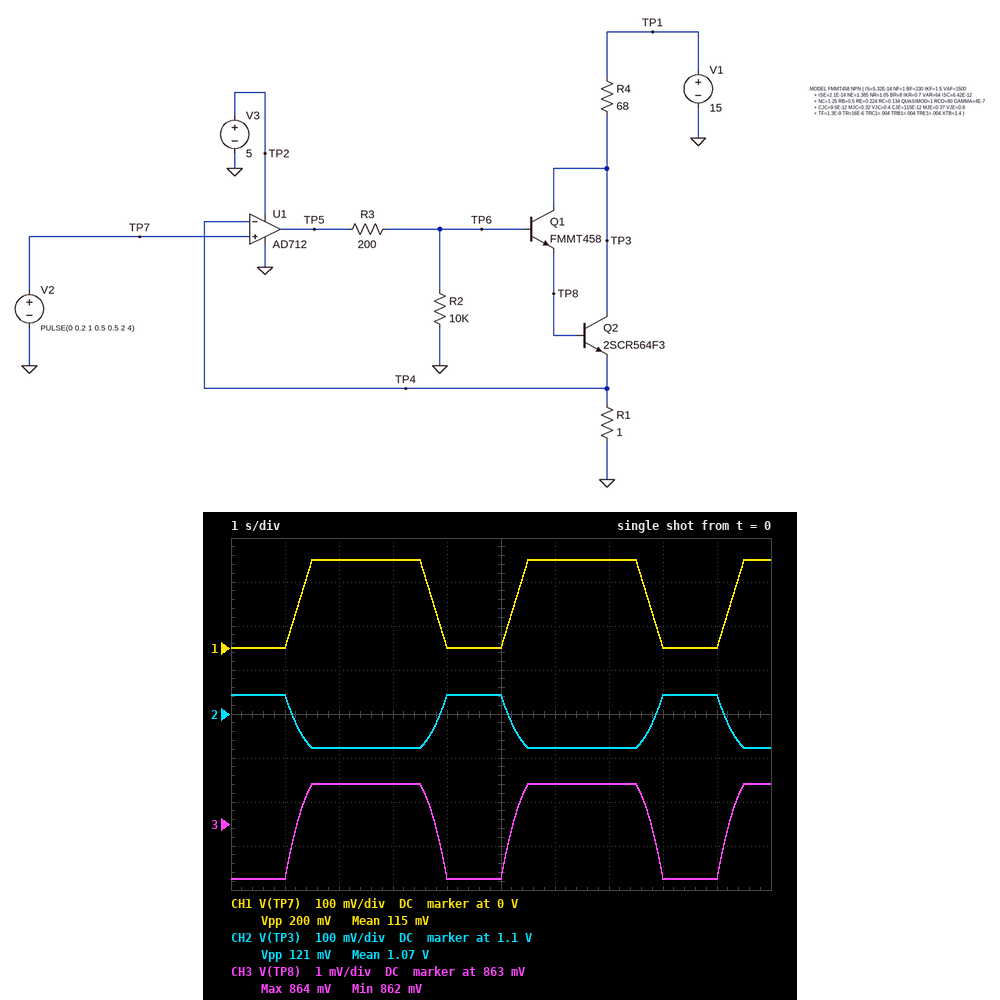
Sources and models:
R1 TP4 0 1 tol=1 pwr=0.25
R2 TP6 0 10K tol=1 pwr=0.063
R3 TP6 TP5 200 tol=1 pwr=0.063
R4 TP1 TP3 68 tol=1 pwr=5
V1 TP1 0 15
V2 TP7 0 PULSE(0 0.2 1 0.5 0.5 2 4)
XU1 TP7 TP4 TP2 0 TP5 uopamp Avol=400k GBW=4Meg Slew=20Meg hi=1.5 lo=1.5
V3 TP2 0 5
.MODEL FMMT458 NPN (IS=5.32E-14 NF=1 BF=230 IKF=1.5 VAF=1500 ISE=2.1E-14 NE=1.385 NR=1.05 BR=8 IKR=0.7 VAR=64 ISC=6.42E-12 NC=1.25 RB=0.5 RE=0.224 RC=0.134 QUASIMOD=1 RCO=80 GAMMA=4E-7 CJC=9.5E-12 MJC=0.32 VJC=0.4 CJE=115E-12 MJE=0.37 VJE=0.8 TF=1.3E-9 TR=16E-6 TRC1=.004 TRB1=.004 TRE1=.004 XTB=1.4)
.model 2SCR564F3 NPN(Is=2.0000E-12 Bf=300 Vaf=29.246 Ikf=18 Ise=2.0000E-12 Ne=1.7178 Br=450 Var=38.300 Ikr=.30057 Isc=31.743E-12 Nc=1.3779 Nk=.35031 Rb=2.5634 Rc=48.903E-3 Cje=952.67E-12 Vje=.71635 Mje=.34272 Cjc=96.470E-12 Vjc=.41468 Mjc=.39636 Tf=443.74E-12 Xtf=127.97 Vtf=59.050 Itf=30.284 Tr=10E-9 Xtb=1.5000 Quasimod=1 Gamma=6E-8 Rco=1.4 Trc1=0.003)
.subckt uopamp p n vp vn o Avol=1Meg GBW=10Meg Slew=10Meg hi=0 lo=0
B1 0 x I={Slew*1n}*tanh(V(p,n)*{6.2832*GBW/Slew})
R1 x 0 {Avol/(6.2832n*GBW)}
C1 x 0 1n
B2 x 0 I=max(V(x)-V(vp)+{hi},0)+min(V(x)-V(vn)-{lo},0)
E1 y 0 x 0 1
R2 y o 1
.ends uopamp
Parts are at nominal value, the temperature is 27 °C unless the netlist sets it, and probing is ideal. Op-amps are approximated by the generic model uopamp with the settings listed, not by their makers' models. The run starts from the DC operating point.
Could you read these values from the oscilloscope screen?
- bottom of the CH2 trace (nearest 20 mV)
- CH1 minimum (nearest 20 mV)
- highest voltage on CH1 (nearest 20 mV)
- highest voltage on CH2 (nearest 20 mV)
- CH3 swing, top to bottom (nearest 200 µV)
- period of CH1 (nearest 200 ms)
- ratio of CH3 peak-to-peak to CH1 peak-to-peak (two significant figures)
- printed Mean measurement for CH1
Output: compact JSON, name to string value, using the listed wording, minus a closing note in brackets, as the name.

{"bottom of the CH2 trace": "1.02 V", "CH1 minimum": "0 V", "highest voltage on CH1": "200 mV", "highest voltage on CH2": "1.14 V", "CH3 swing, top to bottom": "2.2 mV", "period of CH1": "4.0 s", "ratio of CH3 peak-to-peak to CH1 peak-to-peak": "0.011", "printed Mean measurement for CH1": "115 mV"}
